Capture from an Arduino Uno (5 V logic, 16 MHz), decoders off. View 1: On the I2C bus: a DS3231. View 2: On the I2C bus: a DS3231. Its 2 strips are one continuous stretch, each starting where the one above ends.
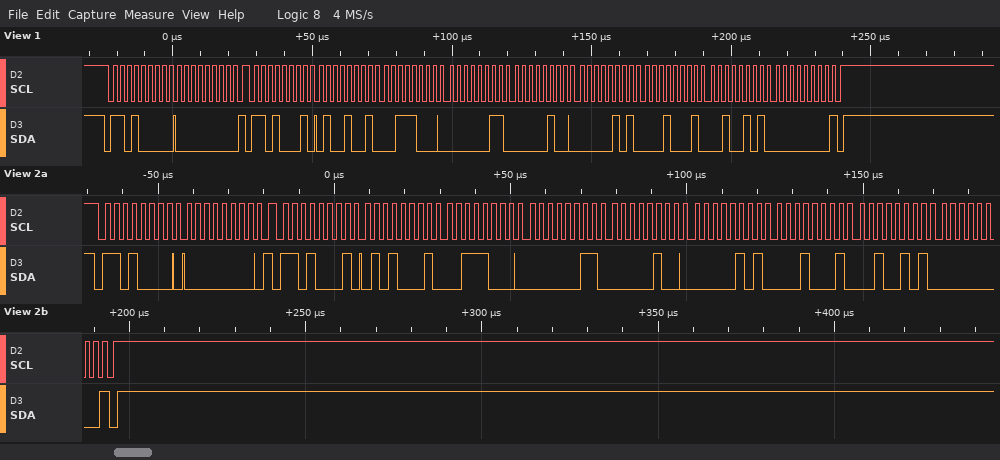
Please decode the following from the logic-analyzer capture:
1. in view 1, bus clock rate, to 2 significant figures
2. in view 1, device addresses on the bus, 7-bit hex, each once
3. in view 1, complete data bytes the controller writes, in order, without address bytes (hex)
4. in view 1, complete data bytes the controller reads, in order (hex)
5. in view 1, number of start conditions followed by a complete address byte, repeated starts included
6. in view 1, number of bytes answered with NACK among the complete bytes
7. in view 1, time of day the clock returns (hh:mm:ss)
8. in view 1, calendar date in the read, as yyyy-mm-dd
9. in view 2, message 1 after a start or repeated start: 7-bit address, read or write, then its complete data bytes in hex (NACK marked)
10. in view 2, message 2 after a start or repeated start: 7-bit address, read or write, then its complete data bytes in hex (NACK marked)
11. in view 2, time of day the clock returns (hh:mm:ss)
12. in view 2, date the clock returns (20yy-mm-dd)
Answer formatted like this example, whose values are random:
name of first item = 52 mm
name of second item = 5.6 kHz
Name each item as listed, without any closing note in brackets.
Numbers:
in view 1, bus clock rate, to 2 significant figures = 400 kHz
in view 1, device addresses on the bus, 7-bit hex, each once = 0x68
in view 1, complete data bytes the controller writes, in order, without address bytes = 00
in view 1, complete data bytes the controller reads, in order = 49 38 03 04 05 11 25 00
in view 1, number of start conditions followed by a complete address byte, repeated starts included = 2
in view 1, number of bytes answered with NACK among the complete bytes = 1
in view 1, time of day the clock returns = 03:38:49
in view 1, calendar date in the read, as yyyy-mm-dd = 2025-11-05
in view 2, message 1 after a start or repeated start: 7-bit address, read or write, then its complete data bytes in hex = 0x68 write: 00
in view 2, message 2 after a start or repeated start: 7-bit address, read or write, then its complete data bytes in hex = 0x68 read: 51 38 03 04 05 11 25 00 NACK
in view 2, time of day the clock returns = 03:38:51
in view 2, date the clock returns = 2025-11-05
